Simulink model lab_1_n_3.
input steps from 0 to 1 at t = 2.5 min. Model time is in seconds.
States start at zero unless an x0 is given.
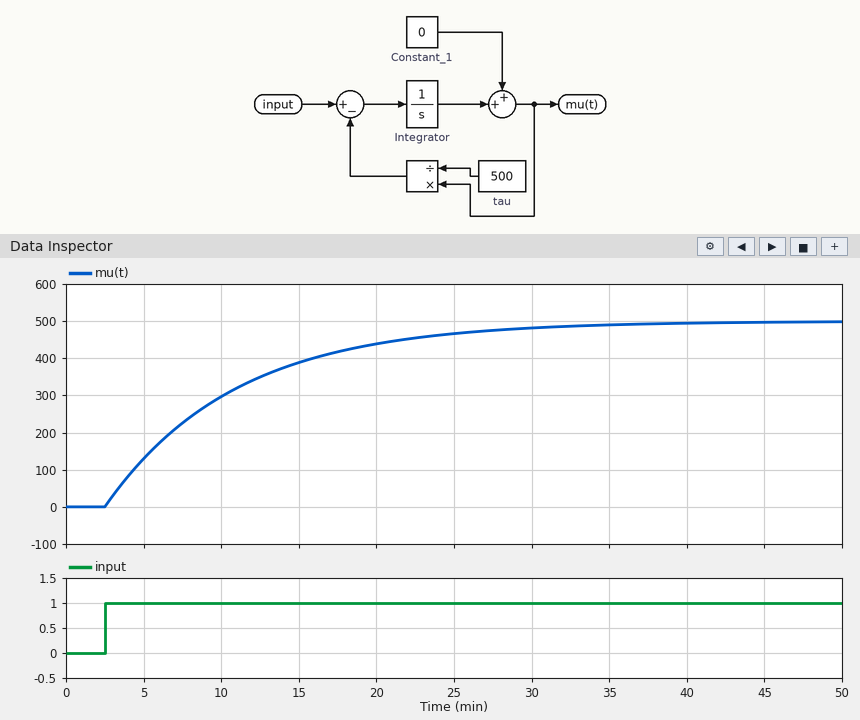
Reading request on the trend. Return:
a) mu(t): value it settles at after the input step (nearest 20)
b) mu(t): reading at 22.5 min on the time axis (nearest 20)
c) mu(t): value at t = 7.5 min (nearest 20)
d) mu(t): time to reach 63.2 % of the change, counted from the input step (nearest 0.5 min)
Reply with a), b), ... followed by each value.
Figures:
a) 500
b) 460
c) 220
d) 8.5 min
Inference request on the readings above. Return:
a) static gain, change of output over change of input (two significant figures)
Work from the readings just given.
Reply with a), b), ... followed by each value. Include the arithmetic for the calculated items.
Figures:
a) (500 - 0) / (1 - 0) = 500
